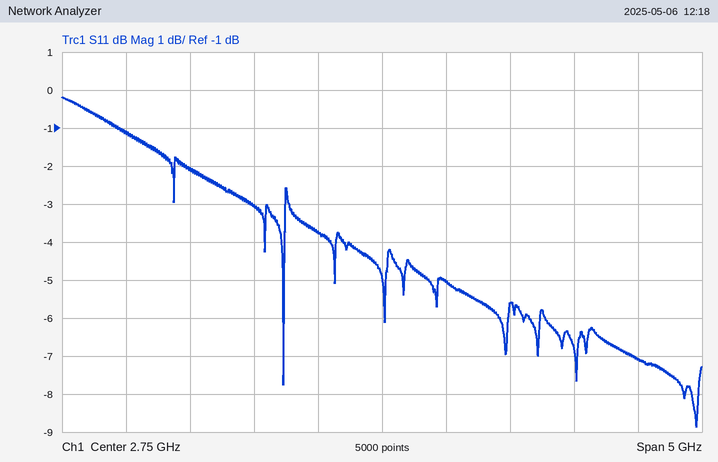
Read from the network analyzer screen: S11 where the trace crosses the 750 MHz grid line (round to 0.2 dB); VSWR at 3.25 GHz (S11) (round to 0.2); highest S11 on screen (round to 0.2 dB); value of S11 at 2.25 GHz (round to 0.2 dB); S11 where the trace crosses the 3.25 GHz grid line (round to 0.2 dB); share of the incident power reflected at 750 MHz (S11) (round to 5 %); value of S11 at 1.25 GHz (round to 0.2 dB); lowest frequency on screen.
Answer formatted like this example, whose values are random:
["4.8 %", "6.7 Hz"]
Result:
["-1.2 dB", "3.6", "-0.2 dB", "-3.8 dB", "-5.0 dB", "75 %", "-2.0 dB", "250 MHz"]
